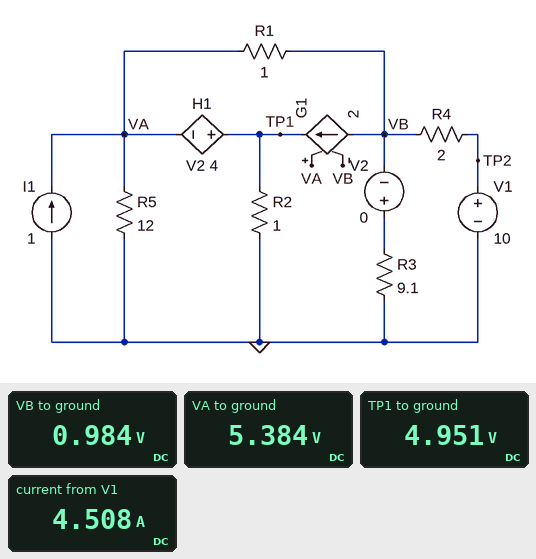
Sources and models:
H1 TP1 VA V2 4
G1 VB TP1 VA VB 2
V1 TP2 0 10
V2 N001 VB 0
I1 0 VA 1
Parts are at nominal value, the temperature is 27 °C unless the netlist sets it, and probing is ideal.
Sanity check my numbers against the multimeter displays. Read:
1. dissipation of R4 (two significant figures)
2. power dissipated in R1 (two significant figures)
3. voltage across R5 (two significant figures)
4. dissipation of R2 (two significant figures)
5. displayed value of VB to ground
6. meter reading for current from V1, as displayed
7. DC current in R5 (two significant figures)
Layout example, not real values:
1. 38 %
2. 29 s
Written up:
1. 41 W
2. 19 W
3. 5.4 V
4. 25 W
5. 0.984 V
6. 4.508 A
7. 450 mA
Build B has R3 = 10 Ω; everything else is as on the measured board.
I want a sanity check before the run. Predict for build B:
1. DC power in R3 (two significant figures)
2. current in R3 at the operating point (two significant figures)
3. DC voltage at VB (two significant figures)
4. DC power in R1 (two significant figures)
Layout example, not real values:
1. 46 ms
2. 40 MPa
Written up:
1. 85 mW
2. 92 mA
3. 920 mV
4. 20 W
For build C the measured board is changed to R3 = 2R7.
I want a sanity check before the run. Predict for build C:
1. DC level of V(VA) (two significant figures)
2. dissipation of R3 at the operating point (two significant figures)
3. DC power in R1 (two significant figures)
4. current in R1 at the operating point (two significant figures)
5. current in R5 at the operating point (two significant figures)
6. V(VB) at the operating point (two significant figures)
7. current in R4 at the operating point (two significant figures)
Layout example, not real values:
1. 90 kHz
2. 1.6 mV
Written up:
1. 4.8 V
2. 570 mW
3. 37 W
4. 6.1 A
5. 400 mA
6. -1.2 V
7. 5.6 A
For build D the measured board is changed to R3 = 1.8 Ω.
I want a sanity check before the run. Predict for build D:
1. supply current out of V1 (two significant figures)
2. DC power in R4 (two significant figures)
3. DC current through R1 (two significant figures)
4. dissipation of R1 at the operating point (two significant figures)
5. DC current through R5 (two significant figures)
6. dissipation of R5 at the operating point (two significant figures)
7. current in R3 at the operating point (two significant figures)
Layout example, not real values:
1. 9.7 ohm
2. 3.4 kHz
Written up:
1. 5.2 A
2. 55 W
3. 5.5 A
4. 30 W
5. 420 mA
6. 2.1 W
7. 260 mA
